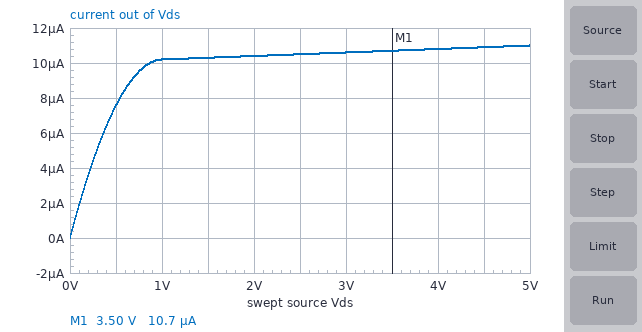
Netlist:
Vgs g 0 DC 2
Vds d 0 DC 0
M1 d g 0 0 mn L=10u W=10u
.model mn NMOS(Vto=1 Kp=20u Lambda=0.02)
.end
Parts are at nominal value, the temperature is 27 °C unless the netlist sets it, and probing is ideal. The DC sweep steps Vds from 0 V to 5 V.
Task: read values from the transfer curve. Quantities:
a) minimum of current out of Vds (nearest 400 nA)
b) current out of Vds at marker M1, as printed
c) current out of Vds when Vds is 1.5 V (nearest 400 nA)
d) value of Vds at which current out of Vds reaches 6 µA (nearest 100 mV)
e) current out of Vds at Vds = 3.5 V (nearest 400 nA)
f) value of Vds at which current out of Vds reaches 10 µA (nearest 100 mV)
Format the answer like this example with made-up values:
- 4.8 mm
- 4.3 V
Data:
- 0 A
- 10.7 µA
- 10.4 µA
- 400 mV
- 10.8 µA
- 900 mV
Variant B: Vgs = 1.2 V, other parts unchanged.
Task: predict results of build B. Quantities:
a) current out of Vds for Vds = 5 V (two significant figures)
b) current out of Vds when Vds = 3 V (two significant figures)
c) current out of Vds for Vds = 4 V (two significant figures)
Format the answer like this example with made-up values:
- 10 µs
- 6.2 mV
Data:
- 440 nA
- 420 nA
- 430 nA
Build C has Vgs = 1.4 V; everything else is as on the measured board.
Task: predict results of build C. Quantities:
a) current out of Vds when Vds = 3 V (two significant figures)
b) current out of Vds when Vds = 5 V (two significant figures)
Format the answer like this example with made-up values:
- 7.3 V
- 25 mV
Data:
- 1.7 µA
- 1.8 µA
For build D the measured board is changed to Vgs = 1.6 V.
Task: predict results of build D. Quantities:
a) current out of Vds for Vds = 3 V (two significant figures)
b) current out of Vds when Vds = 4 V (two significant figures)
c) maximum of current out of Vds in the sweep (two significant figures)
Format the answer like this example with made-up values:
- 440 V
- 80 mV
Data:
- 3.8 µA
- 3.9 µA
- 4.0 µA
